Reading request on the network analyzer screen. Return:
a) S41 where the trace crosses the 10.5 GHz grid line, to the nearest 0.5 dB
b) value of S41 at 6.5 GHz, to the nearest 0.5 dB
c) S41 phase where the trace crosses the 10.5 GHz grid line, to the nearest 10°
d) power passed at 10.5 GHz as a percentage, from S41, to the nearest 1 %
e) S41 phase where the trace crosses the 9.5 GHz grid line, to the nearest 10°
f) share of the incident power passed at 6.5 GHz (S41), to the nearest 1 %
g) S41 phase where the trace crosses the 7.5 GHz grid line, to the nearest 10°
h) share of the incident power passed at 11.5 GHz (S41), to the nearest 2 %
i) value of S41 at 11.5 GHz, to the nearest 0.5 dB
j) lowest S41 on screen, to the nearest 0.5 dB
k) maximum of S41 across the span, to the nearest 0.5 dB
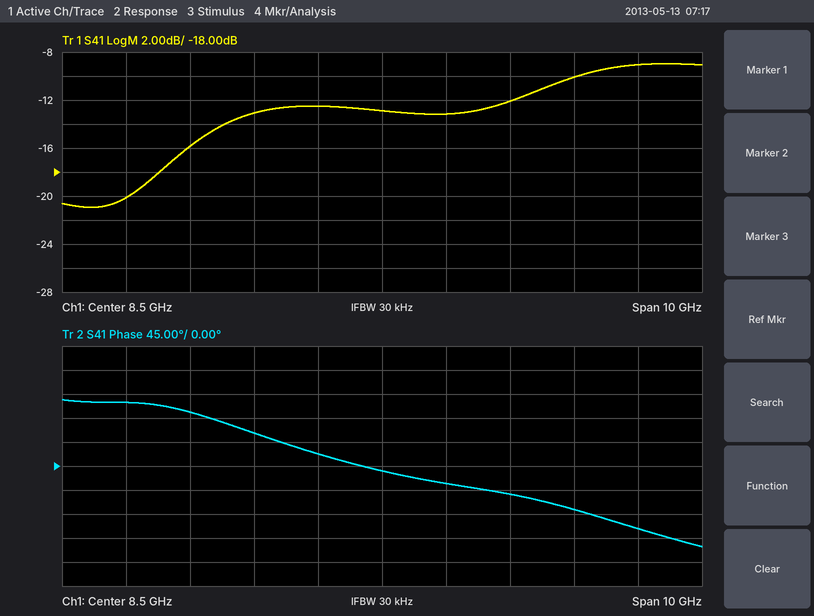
-12.0 dB
-13.0 dB
-50°
6 %
-30°
5 %
20°
10 %
-10.0 dB
-21.0 dB
-9.0 dB
